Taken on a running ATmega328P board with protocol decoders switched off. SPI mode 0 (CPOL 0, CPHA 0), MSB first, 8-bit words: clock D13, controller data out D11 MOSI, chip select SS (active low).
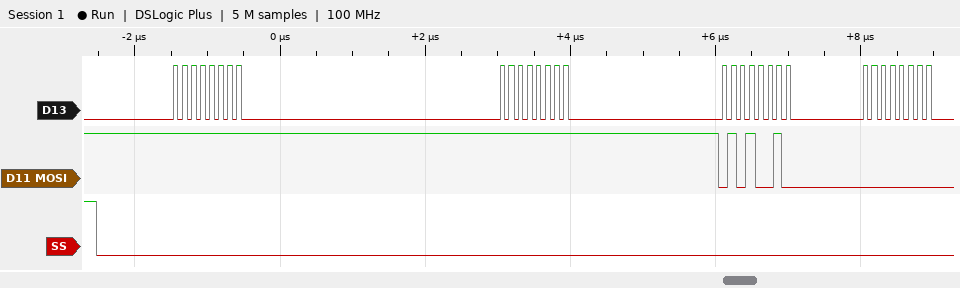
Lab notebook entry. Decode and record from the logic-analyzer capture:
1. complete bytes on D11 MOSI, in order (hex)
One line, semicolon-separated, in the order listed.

0xFF 0xFF 0x52 0x00
